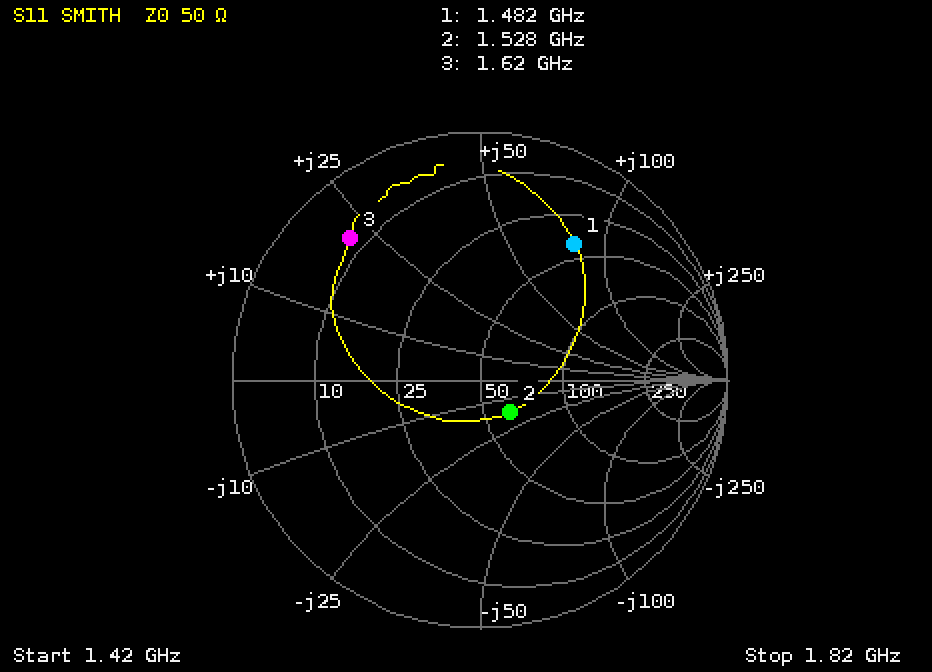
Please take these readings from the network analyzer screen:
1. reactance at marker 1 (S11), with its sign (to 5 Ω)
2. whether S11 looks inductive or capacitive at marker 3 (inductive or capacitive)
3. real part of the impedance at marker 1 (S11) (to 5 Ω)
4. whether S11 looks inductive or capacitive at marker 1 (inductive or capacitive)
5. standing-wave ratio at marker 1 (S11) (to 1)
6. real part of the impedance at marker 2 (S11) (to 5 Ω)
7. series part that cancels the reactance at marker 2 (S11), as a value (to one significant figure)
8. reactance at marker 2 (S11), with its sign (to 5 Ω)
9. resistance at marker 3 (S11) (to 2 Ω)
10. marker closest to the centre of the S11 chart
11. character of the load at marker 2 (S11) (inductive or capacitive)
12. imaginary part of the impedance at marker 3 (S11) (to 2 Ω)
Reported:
+80 Ω
inductive
40 Ω
inductive
5
60 Ω
2 nH
-15 Ω
8 Ω
marker 2
capacitive
+22 Ω
